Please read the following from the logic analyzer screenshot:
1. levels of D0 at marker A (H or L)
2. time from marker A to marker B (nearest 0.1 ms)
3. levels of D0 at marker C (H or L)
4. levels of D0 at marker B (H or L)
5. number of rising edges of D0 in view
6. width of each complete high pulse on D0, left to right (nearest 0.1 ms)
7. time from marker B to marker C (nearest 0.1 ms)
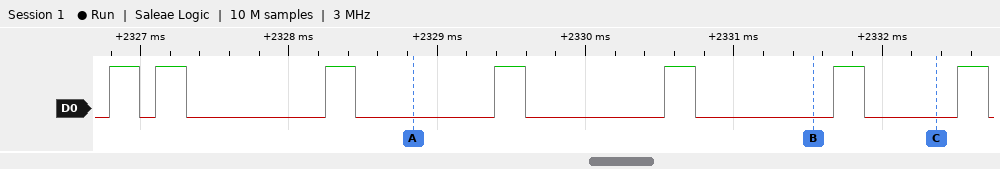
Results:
D0=L
2.7 ms
D0=L
D0=L
7
0.2 ms, 0.2 ms, 0.2 ms, 0.2 ms, 0.2 ms, 0.2 ms, 0.2 ms
0.8 ms
